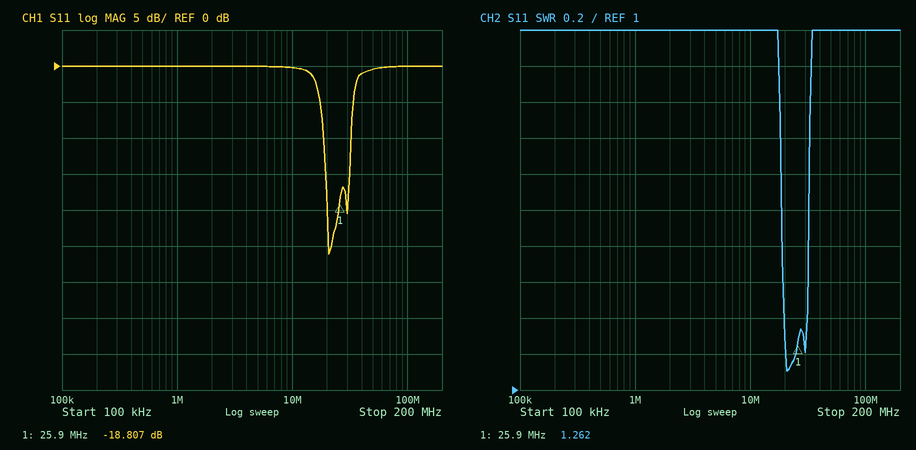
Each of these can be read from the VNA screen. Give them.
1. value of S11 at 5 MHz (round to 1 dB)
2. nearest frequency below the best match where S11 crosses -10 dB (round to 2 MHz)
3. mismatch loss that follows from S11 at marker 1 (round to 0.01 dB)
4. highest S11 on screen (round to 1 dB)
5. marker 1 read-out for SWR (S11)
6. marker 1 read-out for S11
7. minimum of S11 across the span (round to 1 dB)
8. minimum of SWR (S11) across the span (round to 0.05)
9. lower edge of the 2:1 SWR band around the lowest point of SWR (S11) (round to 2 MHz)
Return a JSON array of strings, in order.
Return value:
["0 dB", "18 MHz", "0.06 dB", "0 dB", "1.262", "-18.807 dB", "-26 dB", "1.10", "18 MHz"]
